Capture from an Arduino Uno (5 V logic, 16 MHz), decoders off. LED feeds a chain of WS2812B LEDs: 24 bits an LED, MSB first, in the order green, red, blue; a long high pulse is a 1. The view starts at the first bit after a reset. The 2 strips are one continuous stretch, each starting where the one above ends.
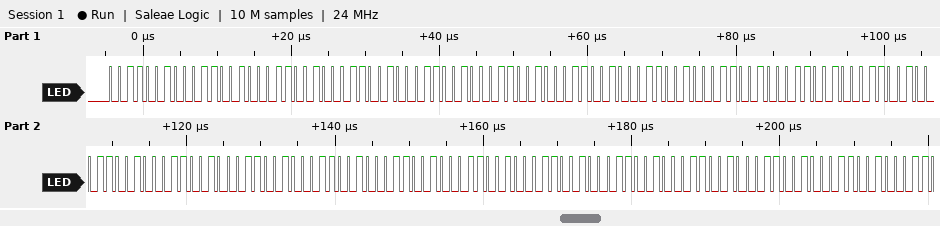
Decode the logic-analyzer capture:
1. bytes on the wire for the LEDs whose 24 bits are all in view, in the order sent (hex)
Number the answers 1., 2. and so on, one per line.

1. 32 32 32 32 32 32 32 32 32 32 32 32 32 32 32 32 32 32 32 32 32
